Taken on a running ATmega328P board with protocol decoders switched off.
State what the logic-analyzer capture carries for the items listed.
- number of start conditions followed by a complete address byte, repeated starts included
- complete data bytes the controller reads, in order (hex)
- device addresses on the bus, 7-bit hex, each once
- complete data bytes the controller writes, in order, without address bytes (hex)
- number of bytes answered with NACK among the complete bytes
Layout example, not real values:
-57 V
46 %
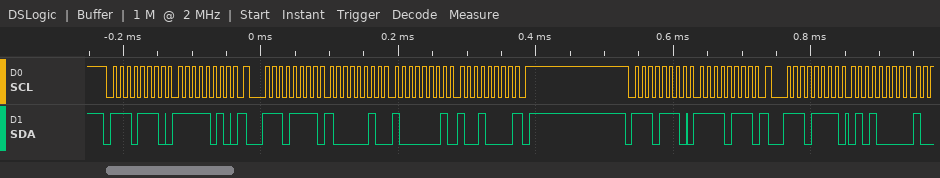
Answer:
4
82 81 90 50
0x77
FA F7
1
